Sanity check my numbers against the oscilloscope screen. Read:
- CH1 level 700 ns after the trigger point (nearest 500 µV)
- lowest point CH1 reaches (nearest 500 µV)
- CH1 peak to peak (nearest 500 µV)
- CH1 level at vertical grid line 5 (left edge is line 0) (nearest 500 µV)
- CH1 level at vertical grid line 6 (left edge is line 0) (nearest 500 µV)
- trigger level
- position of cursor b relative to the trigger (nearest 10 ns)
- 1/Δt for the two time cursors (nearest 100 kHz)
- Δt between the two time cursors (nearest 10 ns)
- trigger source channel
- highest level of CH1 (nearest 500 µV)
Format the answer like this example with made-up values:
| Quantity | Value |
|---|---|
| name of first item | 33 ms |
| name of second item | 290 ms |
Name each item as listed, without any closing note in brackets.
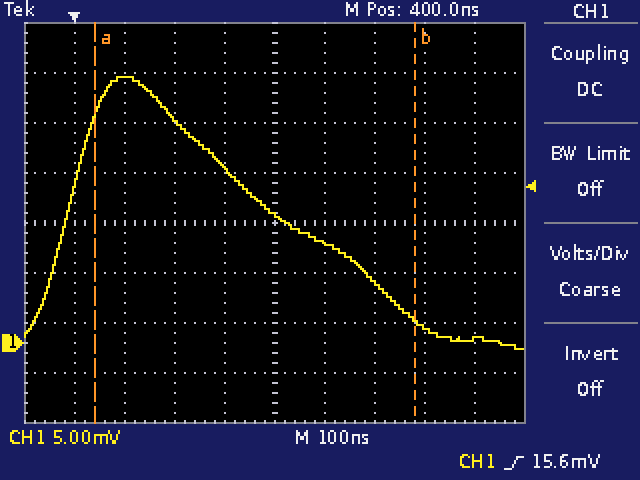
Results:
| Quantity | Value |
|---|---|
| CH1 level 700 ns after the trigger point | 1.5 mV |
| lowest point CH1 reaches | -500 µV |
| CH1 peak to peak | 27.0 mV |
| CH1 level at vertical grid line 5 (left edge is line 0) | 13.0 mV |
| CH1 level at vertical grid line 6 (left edge is line 0) | 10.0 mV |
| trigger level | 15.6 mV |
| position of cursor b relative to the trigger | +680 ns |
| 1/Δt for the two time cursors | 1.6 MHz |
| Δt between the two time cursors | 640 ns |
| trigger source channel | CH1 |
| highest level of CH1 | 26.5 mV |
